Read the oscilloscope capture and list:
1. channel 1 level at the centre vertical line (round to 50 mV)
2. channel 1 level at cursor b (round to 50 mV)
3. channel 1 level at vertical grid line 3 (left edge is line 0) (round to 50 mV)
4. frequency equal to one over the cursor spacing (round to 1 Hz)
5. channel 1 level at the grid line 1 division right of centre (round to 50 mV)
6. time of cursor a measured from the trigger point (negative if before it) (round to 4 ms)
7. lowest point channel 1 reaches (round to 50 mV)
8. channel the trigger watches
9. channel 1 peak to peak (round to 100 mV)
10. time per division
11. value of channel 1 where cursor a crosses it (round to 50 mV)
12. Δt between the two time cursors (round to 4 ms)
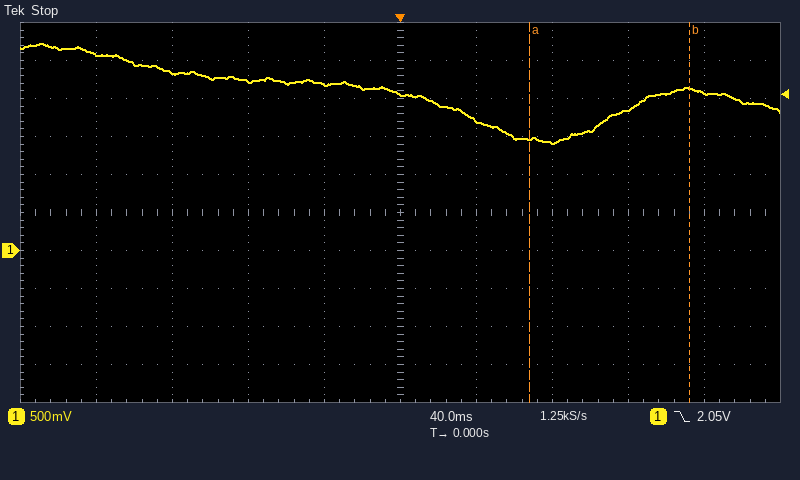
2.05 V
2.15 V
2.25 V
12 Hz
1.70 V
+68 ms
1.40 V
channel 1
1.30 V
40 ms
1.45 V
84 ms
